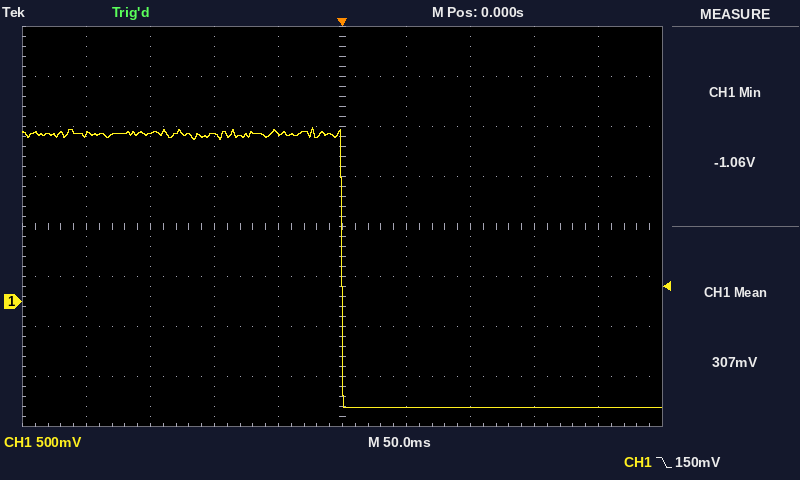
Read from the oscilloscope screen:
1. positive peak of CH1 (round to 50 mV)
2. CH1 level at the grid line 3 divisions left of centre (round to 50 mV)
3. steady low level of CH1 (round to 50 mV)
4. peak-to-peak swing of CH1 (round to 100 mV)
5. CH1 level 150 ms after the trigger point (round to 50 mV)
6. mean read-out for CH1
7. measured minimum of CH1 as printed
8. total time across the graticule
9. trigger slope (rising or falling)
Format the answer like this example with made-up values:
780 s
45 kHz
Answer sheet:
1.75 V
1.70 V
-1.05 V
2.80 V
-1.05 V
307 mV
-1.06 V
500 ms
falling
